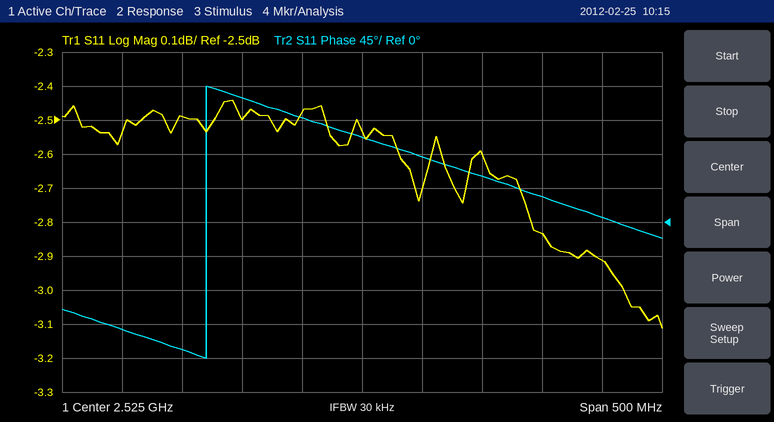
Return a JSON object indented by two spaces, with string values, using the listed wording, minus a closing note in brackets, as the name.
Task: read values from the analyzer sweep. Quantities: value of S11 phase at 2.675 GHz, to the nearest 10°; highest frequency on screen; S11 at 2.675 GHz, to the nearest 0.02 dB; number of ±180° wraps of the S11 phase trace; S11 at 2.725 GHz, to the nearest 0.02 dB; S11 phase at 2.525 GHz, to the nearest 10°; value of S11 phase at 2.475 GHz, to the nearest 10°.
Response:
{
  "value of S11 phase at 2.675 GHz, to the nearest 10°": "30°",
  "highest frequency on screen": "2.775 GHz",
  "S11 at 2.675 GHz, to the nearest 0.02 dB": "-2.84 dB",
  "number of ±180° wraps of the S11 phase trace": "1",
  "S11 at 2.725 GHz, to the nearest 0.02 dB": "-2.92 dB",
  "S11 phase at 2.525 GHz, to the nearest 10°": "110°",
  "value of S11 phase at 2.475 GHz, to the nearest 10°": "140°"
}
